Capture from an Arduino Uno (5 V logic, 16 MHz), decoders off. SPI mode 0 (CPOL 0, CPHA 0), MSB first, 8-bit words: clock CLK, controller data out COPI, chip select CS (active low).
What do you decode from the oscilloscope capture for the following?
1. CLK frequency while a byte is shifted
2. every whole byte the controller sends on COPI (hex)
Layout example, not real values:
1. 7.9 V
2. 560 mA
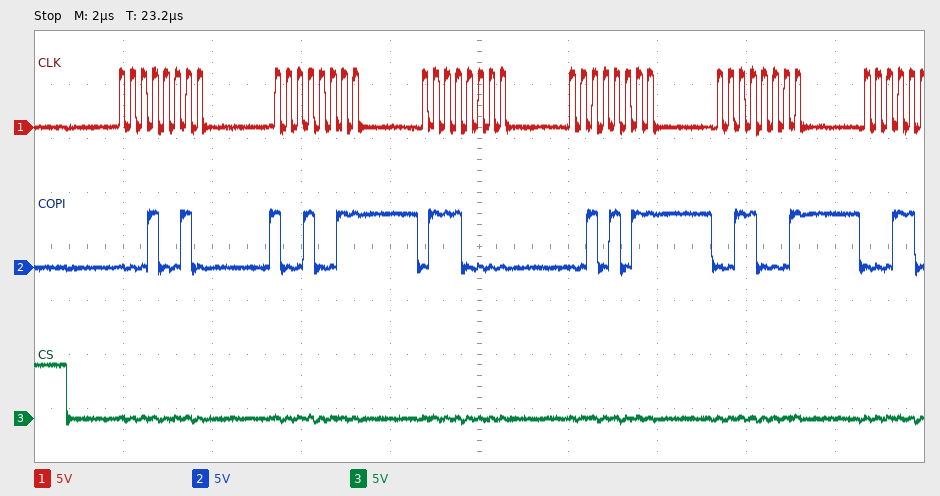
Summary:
1. 4 MHz
2. 12 93 70 2B 31
